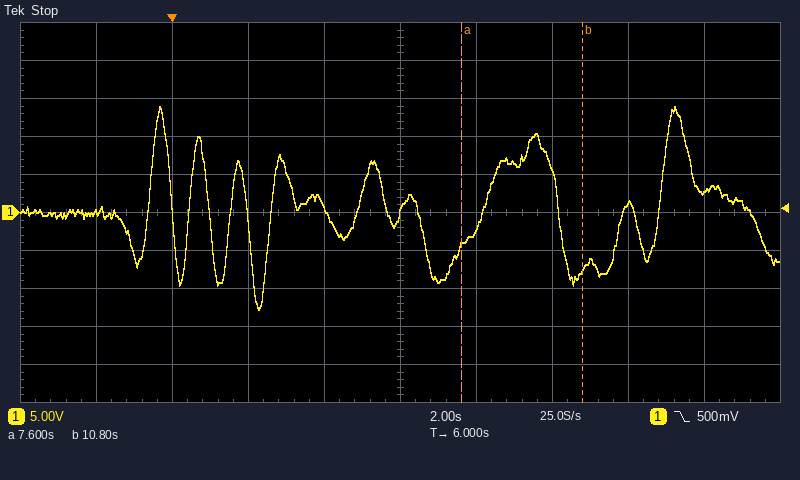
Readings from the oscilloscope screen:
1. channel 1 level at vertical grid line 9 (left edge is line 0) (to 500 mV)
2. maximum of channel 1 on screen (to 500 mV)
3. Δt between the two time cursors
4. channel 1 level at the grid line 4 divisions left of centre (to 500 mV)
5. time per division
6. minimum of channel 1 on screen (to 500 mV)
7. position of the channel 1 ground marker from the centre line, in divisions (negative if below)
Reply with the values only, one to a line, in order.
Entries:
3.0 V
14.0 V
3.2 s
0.0 V
2 s
-13.0 V
0.0 div
